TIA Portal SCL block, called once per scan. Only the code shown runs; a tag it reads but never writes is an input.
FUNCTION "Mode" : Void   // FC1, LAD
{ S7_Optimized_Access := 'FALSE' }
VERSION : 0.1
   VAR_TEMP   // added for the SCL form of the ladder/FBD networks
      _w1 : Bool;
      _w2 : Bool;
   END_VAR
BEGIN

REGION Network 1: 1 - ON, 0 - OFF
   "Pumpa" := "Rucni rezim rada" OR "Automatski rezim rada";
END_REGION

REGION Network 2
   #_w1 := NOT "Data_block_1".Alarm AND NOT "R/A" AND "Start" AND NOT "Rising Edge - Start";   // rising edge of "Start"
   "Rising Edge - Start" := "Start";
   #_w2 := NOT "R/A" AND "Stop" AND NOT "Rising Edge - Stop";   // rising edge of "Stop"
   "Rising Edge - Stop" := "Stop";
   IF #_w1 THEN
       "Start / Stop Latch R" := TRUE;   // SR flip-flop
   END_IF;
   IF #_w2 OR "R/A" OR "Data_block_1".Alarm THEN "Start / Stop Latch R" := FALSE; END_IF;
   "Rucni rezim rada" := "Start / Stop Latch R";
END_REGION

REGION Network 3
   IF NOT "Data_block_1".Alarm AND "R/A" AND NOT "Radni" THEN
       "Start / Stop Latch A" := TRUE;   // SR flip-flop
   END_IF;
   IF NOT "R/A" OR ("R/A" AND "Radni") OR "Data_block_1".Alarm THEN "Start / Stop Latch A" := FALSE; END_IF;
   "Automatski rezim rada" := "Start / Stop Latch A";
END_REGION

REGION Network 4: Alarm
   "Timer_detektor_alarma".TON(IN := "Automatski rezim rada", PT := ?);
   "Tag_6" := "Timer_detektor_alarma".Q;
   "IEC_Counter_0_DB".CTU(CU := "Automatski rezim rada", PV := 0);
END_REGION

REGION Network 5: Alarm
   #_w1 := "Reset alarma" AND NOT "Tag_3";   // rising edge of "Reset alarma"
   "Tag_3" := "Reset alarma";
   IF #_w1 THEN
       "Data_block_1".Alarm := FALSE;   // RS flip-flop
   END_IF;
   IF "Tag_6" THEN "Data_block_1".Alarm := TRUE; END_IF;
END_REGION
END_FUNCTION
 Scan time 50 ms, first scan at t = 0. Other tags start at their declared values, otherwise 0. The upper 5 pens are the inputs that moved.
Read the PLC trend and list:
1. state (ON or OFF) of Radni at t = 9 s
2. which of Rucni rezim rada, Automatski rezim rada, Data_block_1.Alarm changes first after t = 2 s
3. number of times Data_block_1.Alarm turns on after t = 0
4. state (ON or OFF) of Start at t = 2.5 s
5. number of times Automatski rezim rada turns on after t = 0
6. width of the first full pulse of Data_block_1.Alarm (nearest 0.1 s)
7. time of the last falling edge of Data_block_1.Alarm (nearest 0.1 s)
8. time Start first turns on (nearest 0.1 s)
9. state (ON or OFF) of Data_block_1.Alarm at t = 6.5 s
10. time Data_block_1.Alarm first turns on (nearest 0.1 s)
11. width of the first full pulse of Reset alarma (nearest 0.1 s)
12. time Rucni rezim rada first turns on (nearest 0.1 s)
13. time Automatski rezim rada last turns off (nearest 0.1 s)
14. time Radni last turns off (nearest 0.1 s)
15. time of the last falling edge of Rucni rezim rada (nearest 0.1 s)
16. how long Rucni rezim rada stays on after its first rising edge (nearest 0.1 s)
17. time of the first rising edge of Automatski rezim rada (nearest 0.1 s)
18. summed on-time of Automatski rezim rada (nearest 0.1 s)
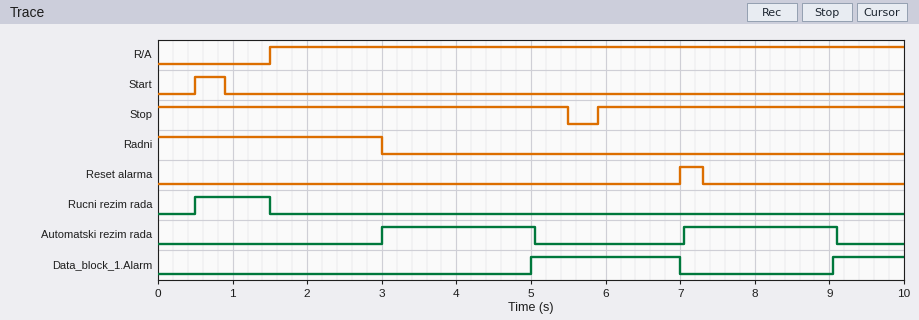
OFF
Automatski rezim rada
2
OFF
2
2.0 s
7.0 s
0.5 s
ON
5.0 s
0.3 s
0.5 s
9.1 s
3.0 s
1.5 s
1.0 s
3.0 s
4.1 s
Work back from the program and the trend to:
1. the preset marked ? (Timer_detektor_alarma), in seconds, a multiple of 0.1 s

2.0 s
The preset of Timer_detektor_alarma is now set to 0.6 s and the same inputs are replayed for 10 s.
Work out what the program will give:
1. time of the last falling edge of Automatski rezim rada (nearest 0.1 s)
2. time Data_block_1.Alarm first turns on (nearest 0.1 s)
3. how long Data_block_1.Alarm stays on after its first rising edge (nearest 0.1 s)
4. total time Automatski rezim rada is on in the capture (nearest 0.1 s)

7.7 s
3.6 s
3.4 s
1.3 s
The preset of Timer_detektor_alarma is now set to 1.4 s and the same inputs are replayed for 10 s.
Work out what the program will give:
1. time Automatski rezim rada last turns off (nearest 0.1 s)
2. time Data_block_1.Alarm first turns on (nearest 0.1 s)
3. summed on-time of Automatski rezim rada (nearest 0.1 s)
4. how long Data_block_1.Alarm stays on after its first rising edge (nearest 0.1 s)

8.5 s
4.4 s
2.9 s
2.6 s
